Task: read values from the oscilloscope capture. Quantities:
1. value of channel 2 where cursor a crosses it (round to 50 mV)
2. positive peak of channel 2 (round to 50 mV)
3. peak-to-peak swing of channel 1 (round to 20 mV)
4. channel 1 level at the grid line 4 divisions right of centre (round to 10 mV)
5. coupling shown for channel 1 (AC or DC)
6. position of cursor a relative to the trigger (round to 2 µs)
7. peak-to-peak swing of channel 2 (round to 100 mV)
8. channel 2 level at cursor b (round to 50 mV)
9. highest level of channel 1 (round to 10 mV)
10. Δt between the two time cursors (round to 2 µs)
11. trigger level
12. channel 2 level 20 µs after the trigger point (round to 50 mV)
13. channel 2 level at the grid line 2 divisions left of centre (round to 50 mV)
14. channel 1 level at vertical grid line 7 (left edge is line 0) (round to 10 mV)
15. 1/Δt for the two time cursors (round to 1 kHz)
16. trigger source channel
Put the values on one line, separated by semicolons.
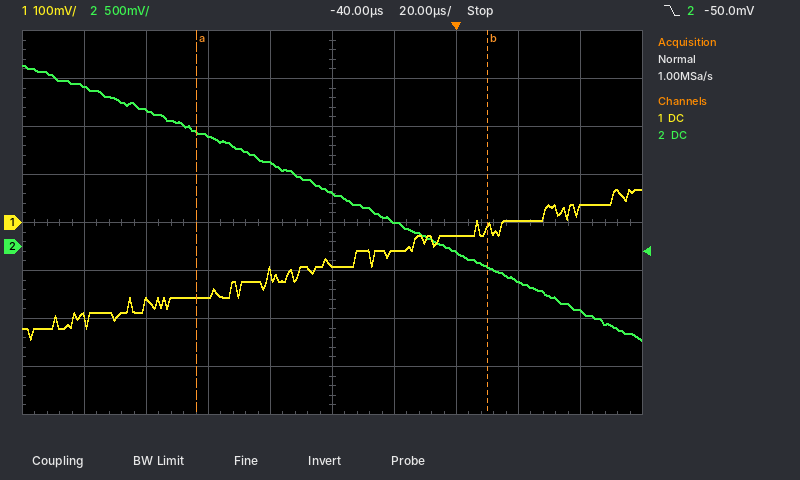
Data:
1.20 V; 1.90 V; 320 mV; 30 mV; DC; -84 µs; 2.90 V; -200 mV; 70 mV; 94 µs; -50.0 mV; -350 mV; 1.15 V; -30 mV; 11 kHz; channel 2
